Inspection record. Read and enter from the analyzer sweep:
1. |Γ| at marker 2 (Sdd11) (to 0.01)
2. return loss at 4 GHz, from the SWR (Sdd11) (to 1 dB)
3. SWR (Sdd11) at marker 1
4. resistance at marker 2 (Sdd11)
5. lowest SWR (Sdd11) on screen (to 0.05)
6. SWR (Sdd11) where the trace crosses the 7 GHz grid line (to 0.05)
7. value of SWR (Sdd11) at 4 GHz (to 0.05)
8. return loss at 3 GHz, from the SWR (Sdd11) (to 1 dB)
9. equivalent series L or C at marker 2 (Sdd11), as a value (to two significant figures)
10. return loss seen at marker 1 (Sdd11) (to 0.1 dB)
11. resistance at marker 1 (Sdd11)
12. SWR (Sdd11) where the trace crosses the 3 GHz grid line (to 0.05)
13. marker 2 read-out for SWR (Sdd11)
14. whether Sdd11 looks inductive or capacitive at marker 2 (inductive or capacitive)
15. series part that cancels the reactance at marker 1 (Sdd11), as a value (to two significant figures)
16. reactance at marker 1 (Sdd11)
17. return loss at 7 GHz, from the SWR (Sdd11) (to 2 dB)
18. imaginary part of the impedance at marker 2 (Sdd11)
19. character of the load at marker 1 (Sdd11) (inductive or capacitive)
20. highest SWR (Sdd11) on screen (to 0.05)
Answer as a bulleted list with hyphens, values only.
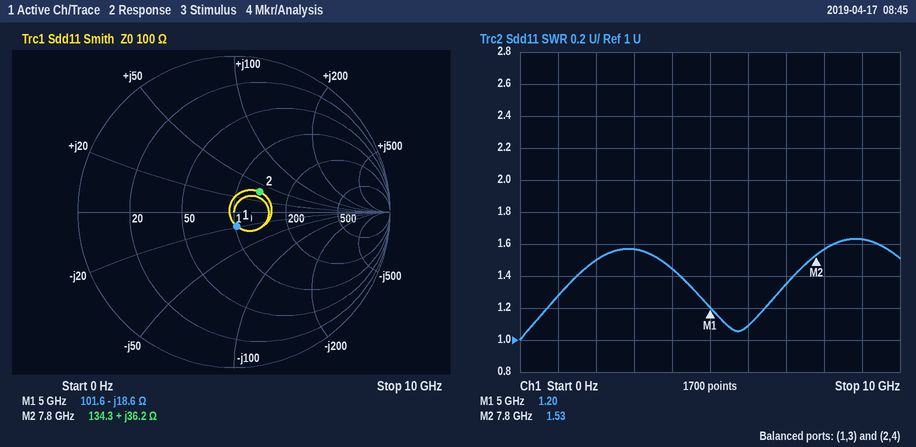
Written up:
- 0.21
- 15 dB
- 1.20
- 134.3 Ω
- 1.00
- 1.35
- 1.45
- 13 dB
- 740 pH
- 20.7 dB
- 101.6 Ω
- 1.55
- 1.53
- inductive
- 590 pH
- -18.6 Ω
- 16 dB
- +36.2 Ω
- capacitive
- 1.65
